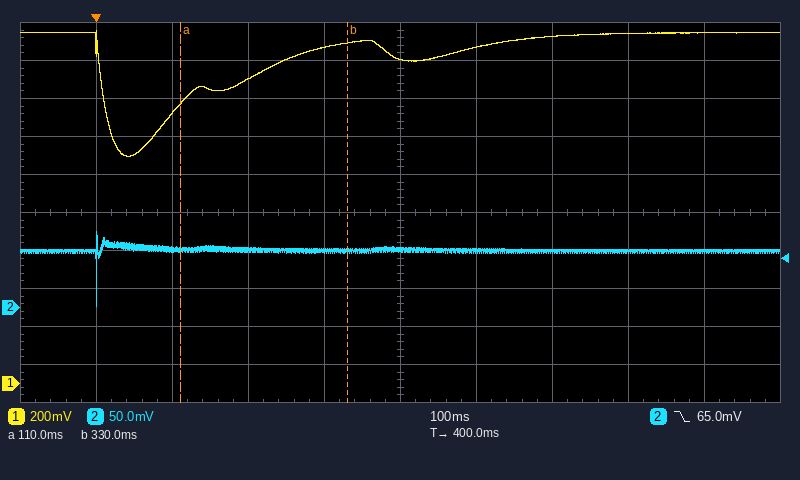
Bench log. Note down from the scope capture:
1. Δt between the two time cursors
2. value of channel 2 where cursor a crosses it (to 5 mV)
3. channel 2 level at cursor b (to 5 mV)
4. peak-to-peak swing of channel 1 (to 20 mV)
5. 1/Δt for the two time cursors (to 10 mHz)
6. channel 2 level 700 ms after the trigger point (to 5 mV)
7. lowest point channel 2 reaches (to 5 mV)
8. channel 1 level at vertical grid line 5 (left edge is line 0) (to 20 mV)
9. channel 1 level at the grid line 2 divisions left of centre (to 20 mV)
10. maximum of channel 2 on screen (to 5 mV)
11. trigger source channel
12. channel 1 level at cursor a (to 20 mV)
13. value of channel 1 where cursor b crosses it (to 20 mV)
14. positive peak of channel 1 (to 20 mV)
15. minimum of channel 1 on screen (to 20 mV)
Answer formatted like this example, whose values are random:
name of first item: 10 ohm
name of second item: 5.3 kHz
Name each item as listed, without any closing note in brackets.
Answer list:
Δt between the two time cursors: 220 ms
value of channel 2 where cursor a crosses it: 75 mV
channel 2 level at cursor b: 75 mV
peak-to-peak swing of channel 1: 660 mV
1/Δt for the two time cursors: 4.55 Hz
channel 2 level 700 ms after the trigger point: 75 mV
lowest point channel 2 reaches: 0 mV
channel 1 level at vertical grid line 5 (left edge is line 0): 1.70 V
channel 1 level at the grid line 2 divisions left of centre: 1.60 V
maximum of channel 2 on screen: 100 mV
trigger source channel: channel 2
channel 1 level at cursor a: 1.48 V
value of channel 1 where cursor b crosses it: 1.80 V
positive peak of channel 1: 1.86 V
minimum of channel 1 on screen: 1.20 V
